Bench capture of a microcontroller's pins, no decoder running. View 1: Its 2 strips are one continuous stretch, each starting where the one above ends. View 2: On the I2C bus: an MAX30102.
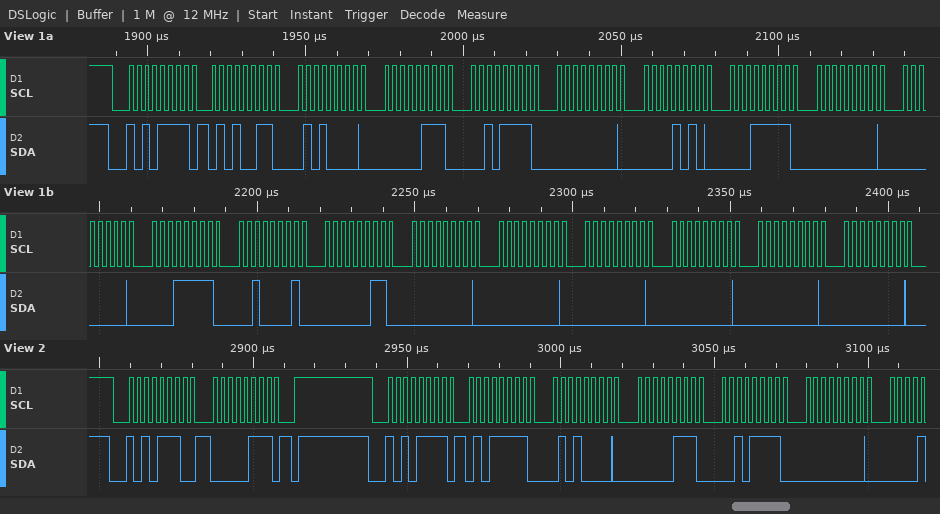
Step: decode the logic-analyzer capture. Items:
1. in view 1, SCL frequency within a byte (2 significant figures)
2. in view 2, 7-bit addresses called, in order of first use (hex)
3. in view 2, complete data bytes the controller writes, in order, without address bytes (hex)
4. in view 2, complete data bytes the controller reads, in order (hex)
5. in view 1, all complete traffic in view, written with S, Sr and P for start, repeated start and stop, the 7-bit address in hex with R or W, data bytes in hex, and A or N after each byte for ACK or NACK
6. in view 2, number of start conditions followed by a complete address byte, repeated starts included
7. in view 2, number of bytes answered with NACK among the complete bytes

400 kHz
0x57
07
5F 50 07 2F 00
S 57R A 53 A 50 A 07 A 2F A 00 A 0A A 1F A 00 A 00 A 1F A 21 A 03 A 00 A 00 A 00 A 00 A 00 A 00 A
2
0
